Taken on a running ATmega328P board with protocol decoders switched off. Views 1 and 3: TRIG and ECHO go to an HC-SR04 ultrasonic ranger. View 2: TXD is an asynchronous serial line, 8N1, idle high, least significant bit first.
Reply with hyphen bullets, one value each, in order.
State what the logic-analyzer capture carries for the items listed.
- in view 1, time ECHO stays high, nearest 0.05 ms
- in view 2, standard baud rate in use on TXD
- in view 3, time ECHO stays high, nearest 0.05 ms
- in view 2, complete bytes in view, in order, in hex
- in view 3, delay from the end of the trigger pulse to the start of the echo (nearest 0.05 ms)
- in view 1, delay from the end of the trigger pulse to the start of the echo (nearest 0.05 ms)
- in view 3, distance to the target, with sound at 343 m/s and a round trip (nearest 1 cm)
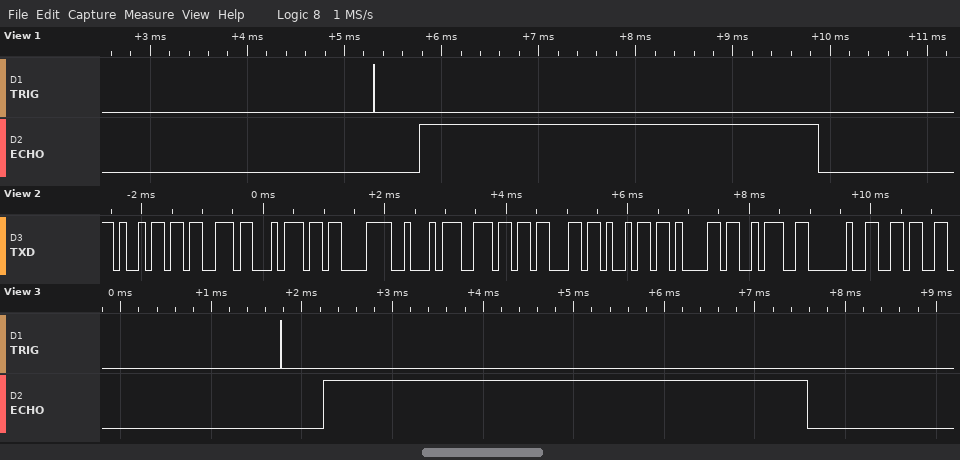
- 4.10 ms
- 9600 baud
- 5.35 ms
- 0x69 0x73 0x74 0xC3 0xA2 0x6E 0x63 0x69 0x61 0x3A 0x20 0x36
- 0.45 ms
- 0.45 ms
- 92 cm
